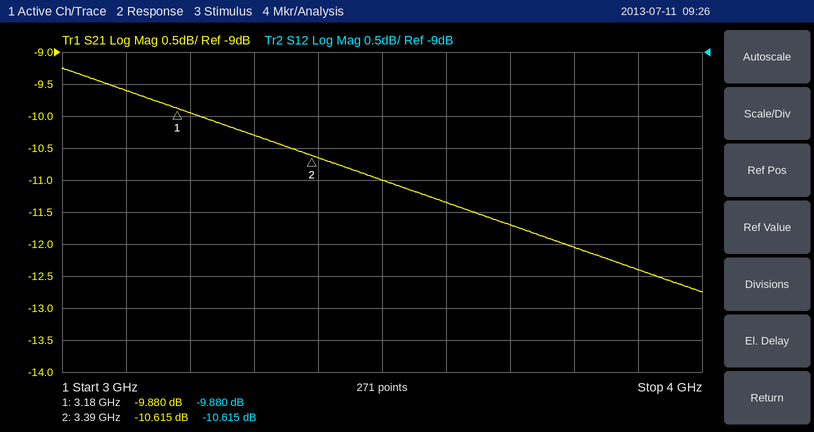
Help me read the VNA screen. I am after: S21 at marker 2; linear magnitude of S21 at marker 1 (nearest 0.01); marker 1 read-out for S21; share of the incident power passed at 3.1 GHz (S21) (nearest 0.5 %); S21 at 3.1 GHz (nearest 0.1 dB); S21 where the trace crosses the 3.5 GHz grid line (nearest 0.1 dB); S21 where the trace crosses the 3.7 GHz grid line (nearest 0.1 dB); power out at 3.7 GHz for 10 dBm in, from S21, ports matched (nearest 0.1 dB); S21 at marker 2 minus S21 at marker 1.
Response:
-10.615 dB
0.32
-9.880 dB
11.0 %
-9.6 dB
-11.0 dB
-11.7 dB
-1.7 dBm
-0.735 dB
